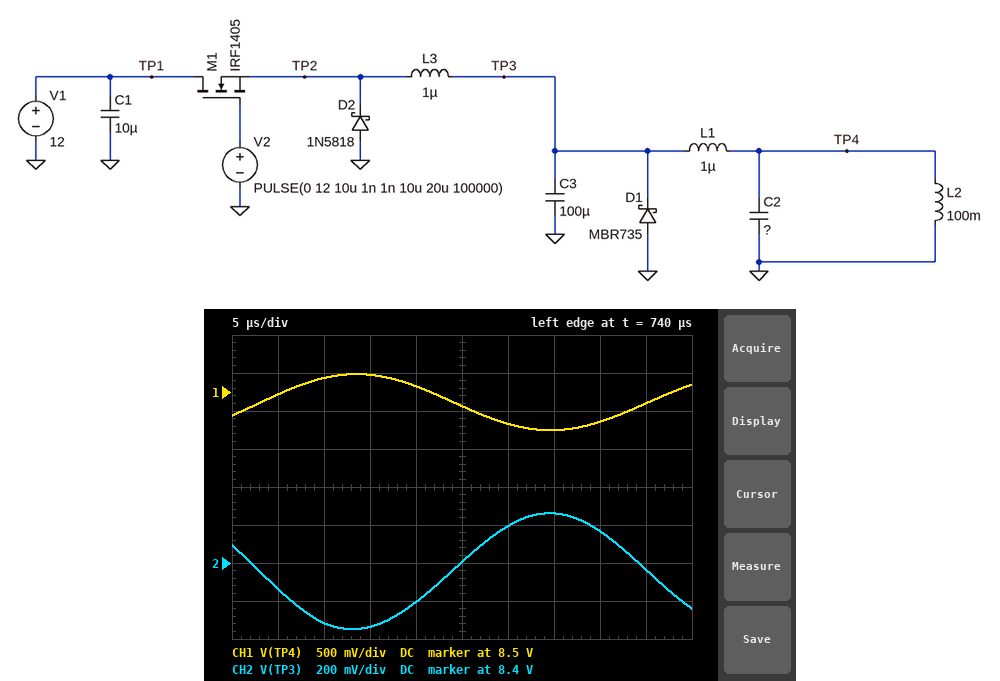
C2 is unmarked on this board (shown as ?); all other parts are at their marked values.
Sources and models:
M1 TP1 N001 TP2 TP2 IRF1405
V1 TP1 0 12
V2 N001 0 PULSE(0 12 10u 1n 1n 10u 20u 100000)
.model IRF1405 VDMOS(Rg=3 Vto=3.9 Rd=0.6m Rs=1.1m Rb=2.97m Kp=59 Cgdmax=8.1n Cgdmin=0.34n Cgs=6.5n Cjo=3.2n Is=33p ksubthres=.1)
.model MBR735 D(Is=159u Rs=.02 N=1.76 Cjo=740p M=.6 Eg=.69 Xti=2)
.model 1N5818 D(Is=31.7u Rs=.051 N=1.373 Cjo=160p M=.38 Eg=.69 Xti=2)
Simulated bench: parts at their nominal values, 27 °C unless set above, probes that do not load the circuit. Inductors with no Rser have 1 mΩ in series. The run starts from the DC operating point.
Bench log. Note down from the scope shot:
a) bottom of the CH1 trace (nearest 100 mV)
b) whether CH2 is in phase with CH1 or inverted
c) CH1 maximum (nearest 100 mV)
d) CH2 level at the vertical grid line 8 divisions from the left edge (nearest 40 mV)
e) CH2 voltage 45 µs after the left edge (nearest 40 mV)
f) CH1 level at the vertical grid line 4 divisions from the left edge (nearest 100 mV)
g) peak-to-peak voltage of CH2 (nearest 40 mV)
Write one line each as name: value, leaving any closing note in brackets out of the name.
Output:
bottom of the CH1 trace: 8.0 V
whether CH2 is in phase with CH1 or inverted: inverted
CH1 maximum: 8.7 V
CH2 level at the vertical grid line 8 divisions from the left edge: 8.56 V
CH2 voltage 45 µs after the left edge: 8.36 V
CH1 level at the vertical grid line 4 divisions from the left edge: 8.6 V
peak-to-peak voltage of CH2: 600 mV
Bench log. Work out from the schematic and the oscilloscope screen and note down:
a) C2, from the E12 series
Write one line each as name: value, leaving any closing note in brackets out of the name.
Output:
C2, from the E12 series: 82 µF
